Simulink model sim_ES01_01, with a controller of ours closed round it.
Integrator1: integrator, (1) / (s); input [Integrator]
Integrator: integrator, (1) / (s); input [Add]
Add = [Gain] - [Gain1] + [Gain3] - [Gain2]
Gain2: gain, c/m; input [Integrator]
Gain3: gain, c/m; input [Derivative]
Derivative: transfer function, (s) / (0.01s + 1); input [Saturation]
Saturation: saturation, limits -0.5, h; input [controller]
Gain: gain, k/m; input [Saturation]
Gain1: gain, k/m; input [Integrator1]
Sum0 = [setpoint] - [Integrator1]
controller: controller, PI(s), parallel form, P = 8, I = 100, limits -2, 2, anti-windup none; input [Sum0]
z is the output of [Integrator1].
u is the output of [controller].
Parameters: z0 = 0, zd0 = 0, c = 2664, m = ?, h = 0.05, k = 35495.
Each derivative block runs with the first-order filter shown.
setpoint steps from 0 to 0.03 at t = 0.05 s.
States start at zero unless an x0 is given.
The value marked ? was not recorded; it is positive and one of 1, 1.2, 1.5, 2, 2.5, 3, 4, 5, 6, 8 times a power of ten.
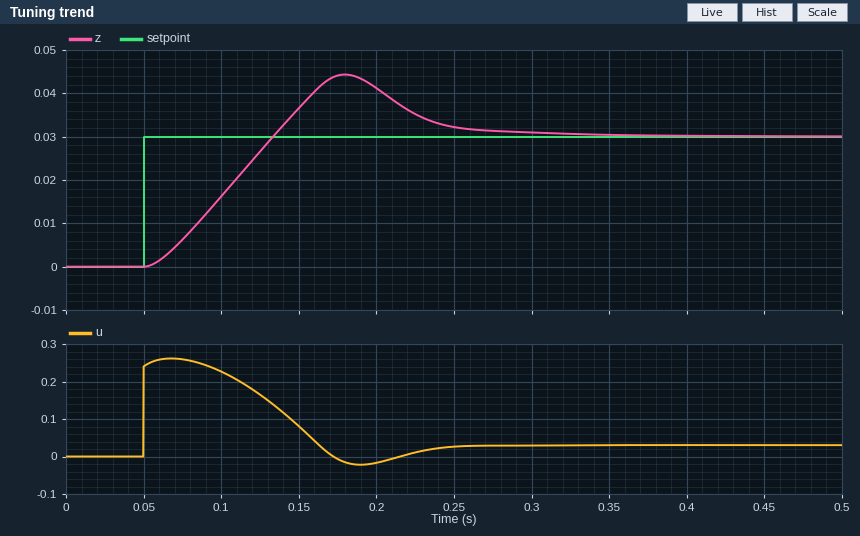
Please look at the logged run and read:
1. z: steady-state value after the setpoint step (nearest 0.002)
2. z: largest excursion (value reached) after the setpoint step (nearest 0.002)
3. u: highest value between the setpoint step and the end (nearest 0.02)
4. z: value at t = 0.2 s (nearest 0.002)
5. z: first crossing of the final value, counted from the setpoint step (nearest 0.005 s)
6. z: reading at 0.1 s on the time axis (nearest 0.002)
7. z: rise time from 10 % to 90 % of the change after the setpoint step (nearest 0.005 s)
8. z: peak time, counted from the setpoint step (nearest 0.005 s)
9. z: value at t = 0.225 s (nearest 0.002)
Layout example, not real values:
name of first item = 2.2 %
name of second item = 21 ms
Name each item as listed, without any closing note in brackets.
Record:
z: steady-state value after the setpoint step = 0.030
z: largest excursion (value reached) after the setpoint step = 0.044
u: highest value between the setpoint step and the end = 0.26
z: value at t = 0.2 s = 0.042
z: first crossing of the final value, counted from the setpoint step = 0.085 s
z: reading at 0.1 s on the time axis = 0.016
z: rise time from 10 % to 90 % of the change after the setpoint step = 0.060 s
z: peak time, counted from the setpoint step = 0.130 s
z: value at t = 0.225 s = 0.036
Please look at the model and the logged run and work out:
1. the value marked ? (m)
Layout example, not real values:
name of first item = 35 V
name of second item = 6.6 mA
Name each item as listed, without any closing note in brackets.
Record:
the value marked ? = 400
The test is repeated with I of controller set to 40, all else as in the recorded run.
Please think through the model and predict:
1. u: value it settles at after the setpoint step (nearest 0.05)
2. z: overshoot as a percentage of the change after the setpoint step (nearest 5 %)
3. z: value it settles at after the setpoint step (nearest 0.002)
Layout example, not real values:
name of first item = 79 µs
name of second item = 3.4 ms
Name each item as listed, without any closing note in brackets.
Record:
u: value it settles at after the setpoint step = 0.05
z: overshoot as a percentage of the change after the setpoint step = 25 %
z: value it settles at after the setpoint step = 0.030
